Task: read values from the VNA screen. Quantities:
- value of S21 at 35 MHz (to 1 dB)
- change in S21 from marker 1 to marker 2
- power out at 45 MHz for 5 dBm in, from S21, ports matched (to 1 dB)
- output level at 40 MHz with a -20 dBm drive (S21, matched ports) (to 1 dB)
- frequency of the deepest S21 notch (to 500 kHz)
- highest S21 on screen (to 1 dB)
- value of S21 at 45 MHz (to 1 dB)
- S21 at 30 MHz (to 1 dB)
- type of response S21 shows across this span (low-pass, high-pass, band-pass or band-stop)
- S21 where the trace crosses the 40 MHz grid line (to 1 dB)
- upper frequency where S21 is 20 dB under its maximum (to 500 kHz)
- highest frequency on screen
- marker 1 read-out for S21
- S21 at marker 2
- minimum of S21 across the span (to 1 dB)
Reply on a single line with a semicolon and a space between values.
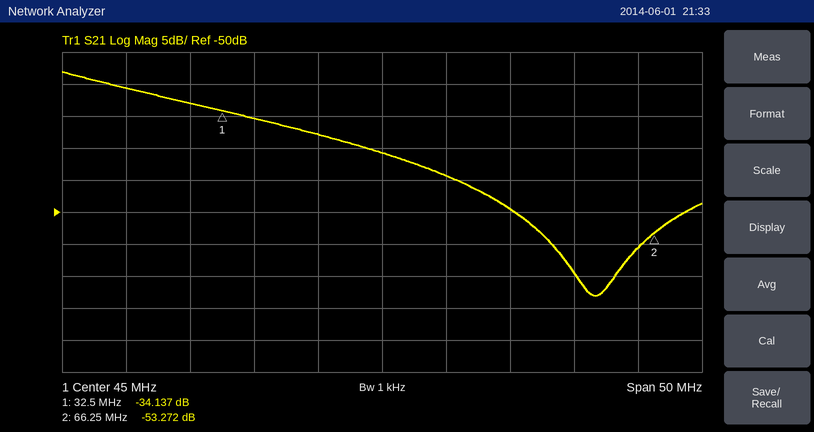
-35 dB; -19.135 dB; -36 dBm; -58 dBm; 61.5 MHz; -28 dB; -41 dB; -33 dB; low-pass; -38 dB; 54.0 MHz; 70 MHz; -34.137 dB; -53.272 dB; -63 dB
